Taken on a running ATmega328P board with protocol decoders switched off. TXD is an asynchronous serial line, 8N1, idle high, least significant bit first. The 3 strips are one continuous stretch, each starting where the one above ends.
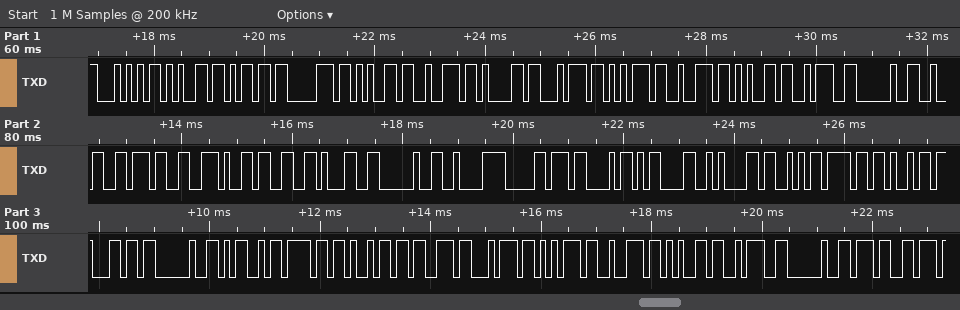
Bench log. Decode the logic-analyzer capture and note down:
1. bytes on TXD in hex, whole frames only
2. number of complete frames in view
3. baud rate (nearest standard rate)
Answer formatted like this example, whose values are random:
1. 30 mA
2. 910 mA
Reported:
1. 54 65 6D 70 65 72 61 74 75 72 65 3A 20 32 37 2E 33 31 20 C2 B0 43 0D 0A 53 6F 69 6C 20 4D 6F 69 73 74 75 72 65 3A 20 37
2. 40
3. 9600 baud
